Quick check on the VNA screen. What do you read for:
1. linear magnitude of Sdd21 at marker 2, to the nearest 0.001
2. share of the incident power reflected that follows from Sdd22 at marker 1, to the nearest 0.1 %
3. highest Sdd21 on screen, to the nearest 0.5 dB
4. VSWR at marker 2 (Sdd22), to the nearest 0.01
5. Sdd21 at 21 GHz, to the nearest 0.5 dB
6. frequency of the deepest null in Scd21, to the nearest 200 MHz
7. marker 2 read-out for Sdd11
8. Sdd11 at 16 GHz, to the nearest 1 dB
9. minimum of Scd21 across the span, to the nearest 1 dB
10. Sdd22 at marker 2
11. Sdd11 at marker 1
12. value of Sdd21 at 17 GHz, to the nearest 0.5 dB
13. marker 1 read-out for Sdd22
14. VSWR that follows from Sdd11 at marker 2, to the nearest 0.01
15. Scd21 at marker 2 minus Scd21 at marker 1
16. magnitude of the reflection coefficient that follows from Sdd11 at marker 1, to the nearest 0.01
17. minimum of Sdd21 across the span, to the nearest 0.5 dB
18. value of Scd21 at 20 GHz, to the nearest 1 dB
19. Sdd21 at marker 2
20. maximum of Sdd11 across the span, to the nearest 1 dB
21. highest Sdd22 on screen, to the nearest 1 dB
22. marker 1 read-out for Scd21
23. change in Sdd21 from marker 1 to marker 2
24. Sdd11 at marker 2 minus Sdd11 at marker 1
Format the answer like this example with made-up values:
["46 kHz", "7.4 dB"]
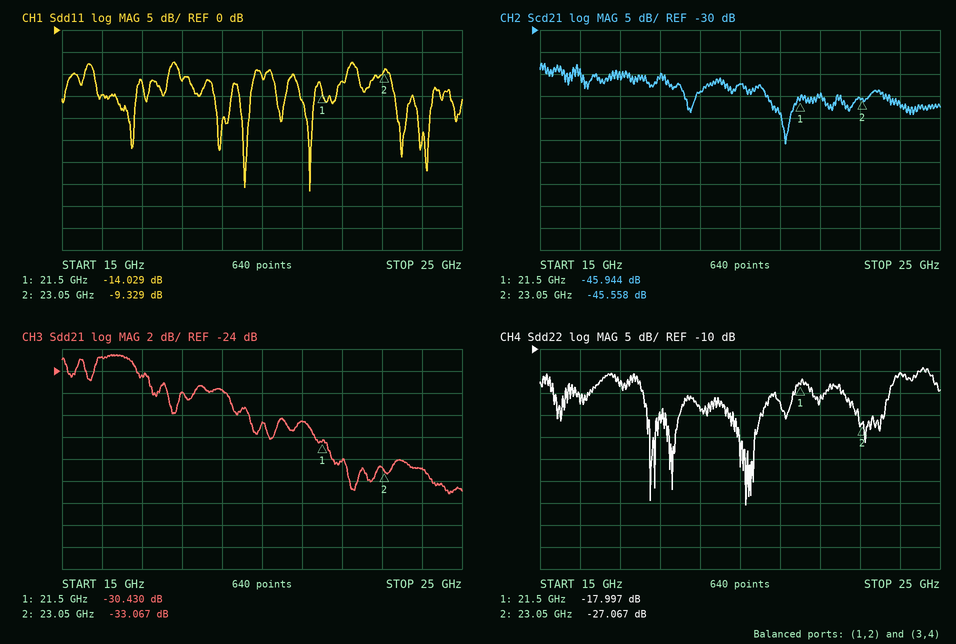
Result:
["0.022", "1.6 %", "-22.5 dB", "1.09", "-28.5 dB", "21.2 GHz", "-9.329 dB", "-15 dB", "-56 dB", "-27.067 dB", "-14.029 dB", "-24.5 dB", "-17.997 dB", "2.04", "0.386 dB", "0.20", "-35.0 dB", "-42 dB", "-33.067 dB", "-7 dB", "-14 dB", "-45.944 dB", "-2.637 dB", "4.700 dB"]
